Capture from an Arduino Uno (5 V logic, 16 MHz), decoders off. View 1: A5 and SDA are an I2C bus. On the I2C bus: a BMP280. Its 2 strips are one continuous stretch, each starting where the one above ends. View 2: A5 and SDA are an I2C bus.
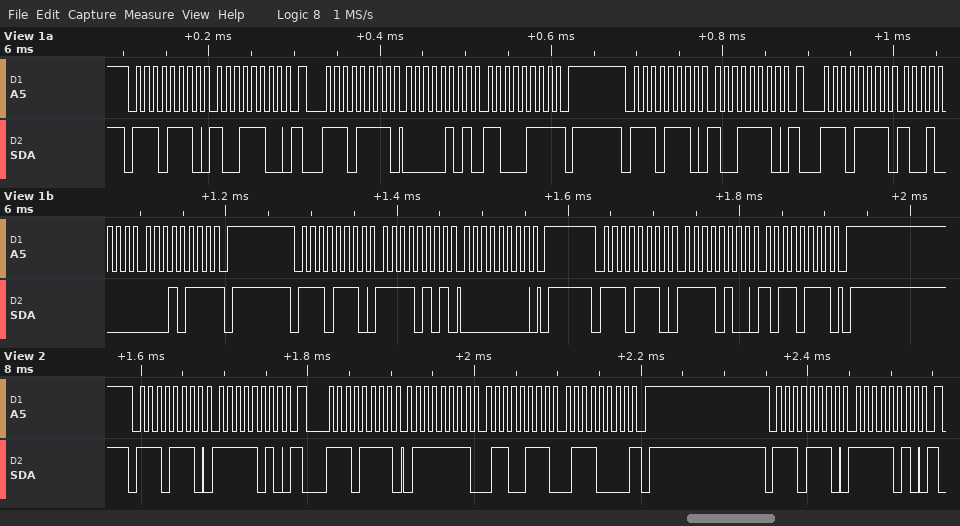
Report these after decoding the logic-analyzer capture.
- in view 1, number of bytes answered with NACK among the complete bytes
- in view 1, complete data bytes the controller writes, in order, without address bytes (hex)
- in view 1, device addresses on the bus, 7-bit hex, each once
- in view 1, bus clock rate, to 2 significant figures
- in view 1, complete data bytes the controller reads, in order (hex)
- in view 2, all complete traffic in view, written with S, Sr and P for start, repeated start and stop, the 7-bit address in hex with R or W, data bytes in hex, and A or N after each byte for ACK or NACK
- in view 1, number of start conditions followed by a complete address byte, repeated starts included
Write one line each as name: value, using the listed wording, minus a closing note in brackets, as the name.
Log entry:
in view 1, number of bytes answered with NACK among the complete bytes: 2
in view 1, complete data bytes the controller writes, in order, without address bytes: 9C 9E F5 00 F4 B7
in view 1, device addresses on the bus, 7-bit hex, each once: 0x77
in view 1, bus clock rate, to 2 significant figures: 100 kHz
in view 1, complete data bytes the controller reads, in order: 05 C7 90 17
in view 2, all complete traffic in view, written with S, Sr and P for start, repeated start and stop, the 7-bit address in hex with R or W, data bytes in hex, and A or N after each byte for ACK or NACK: S 77W A FA A Sr 77R A 7F A 67 A 70 N P S 77W A FA A
in view 1, number of start conditions followed by a complete address byte, repeated starts included: 6
